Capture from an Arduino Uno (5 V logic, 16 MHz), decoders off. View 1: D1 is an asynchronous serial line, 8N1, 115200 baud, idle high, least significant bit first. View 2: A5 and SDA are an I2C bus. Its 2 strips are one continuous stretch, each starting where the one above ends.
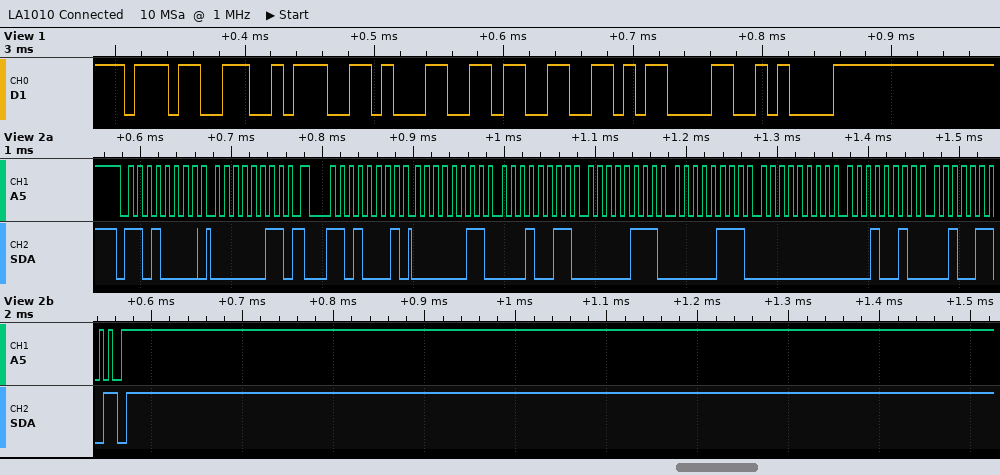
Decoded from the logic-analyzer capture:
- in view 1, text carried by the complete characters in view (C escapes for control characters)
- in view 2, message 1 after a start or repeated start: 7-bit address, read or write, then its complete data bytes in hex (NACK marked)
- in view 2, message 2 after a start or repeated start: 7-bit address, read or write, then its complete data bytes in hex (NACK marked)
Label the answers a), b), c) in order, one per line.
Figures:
a) "7:13\r\n"
b) 0x68 write: 03
c) 0x68 read: 03 13 07 07 00 12 26 NACK
